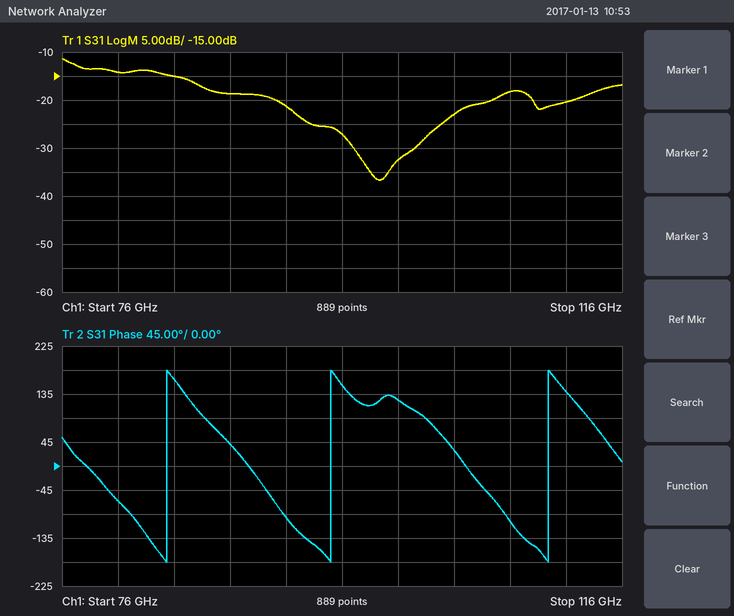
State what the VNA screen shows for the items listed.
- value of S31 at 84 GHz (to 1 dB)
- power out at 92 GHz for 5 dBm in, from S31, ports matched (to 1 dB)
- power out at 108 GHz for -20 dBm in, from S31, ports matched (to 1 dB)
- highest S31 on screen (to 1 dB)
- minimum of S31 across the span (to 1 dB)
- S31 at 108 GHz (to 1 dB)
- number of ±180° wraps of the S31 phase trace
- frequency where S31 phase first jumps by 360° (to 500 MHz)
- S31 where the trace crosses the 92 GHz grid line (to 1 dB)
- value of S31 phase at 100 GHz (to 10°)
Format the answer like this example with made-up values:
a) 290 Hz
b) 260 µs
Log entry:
a) -15 dB
b) -16 dBm
c) -38 dBm
d) -11 dB
e) -37 dB
f) -18 dB
g) 3
h) 83.5 GHz
i) -21 dB
j) 120°
